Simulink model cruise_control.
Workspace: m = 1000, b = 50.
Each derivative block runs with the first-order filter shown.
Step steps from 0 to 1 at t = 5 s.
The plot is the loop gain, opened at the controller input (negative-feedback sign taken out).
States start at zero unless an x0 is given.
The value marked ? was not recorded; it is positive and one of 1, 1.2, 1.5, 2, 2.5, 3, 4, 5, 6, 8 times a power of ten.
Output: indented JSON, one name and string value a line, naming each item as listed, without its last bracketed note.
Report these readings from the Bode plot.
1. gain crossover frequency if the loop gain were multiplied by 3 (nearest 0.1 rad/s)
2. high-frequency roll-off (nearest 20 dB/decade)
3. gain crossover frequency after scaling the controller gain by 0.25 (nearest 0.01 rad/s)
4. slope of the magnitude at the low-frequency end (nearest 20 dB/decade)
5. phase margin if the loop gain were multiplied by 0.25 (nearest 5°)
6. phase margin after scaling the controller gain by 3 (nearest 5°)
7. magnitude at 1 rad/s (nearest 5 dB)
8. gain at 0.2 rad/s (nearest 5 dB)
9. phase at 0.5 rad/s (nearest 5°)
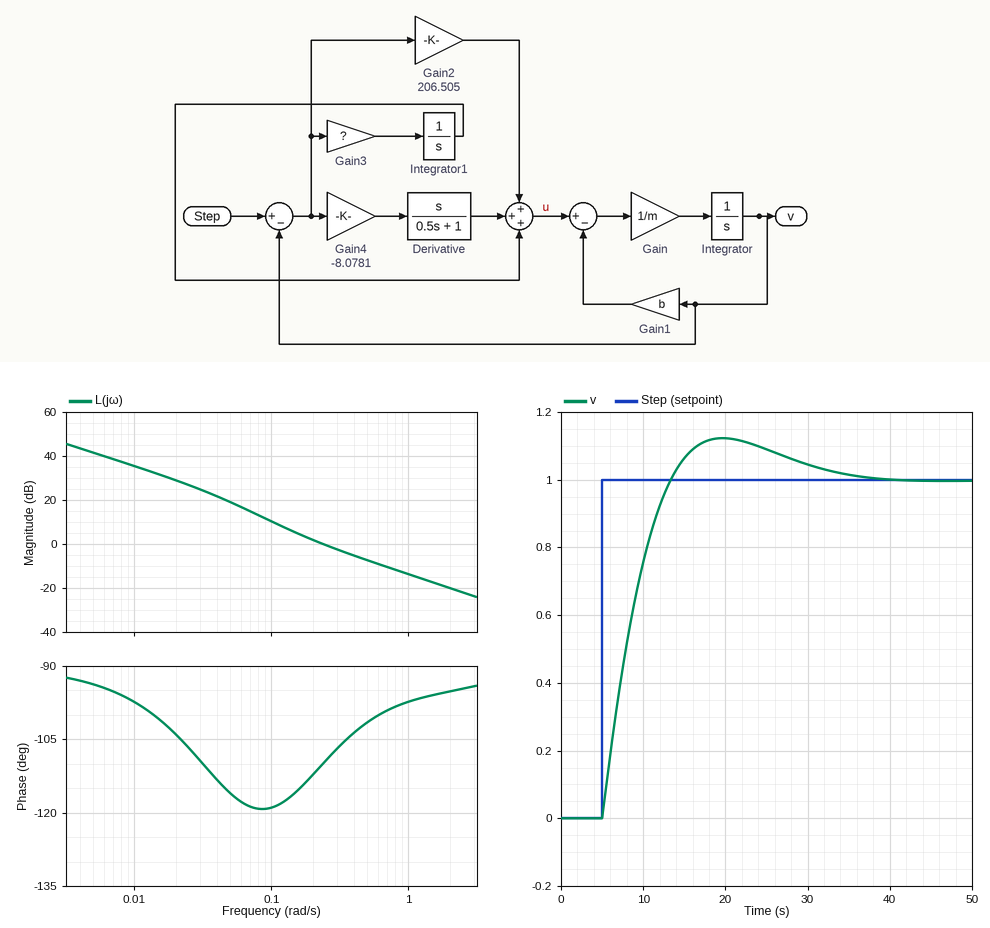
{
  "gain crossover frequency if the loop gain were multiplied by 3": "0.6 rad/s",
  "high-frequency roll-off": "-20 dB/decade",
  "gain crossover frequency after scaling the controller gain by 0.25": "0.09 rad/s",
  "slope of the magnitude at the low-frequency end": "-20 dB/decade",
  "phase margin if the loop gain were multiplied by 0.25": "60°",
  "phase margin after scaling the controller gain by 3": "80°",
  "magnitude at 1 rad/s": "-15 dB",
  "gain at 0.2 rad/s": "0 dB",
  "phase at 0.5 rad/s": "-100°"
}
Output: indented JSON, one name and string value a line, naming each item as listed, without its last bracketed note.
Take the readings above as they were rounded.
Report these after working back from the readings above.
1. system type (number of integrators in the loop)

{
  "system type": "1"
}
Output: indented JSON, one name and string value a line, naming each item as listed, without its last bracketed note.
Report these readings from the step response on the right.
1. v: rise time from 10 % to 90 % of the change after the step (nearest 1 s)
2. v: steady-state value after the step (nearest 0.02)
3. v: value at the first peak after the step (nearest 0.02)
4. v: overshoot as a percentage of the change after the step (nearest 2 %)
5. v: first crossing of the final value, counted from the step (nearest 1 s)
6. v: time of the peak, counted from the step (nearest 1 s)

{
  "v: rise time from 10 % to 90 % of the change after the step": "6 s",
  "v: steady-state value after the step": "1.00",
  "v: value at the first peak after the step": "1.12",
  "v: overshoot as a percentage of the change after the step": "12 %",
  "v: first crossing of the final value, counted from the step": "8 s",
  "v: time of the peak, counted from the step": "15 s"
}
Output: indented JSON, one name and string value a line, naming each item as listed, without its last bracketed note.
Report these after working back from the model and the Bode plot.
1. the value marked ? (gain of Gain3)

{
  "the value marked ?": "30"
}
